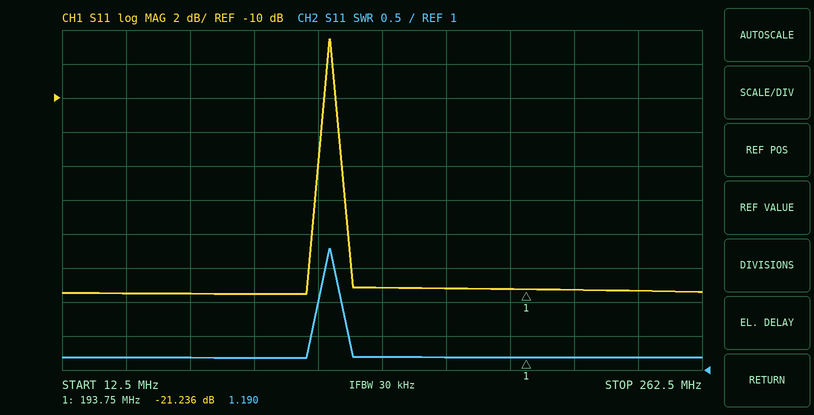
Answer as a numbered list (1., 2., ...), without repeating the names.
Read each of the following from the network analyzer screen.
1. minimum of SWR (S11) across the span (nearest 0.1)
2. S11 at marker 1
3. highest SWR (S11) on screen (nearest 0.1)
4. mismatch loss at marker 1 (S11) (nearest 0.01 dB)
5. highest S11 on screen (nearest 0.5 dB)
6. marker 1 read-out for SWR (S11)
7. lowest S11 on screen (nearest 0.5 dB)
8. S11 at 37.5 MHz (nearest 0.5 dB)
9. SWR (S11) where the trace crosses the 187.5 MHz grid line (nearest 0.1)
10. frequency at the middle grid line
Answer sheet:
1. 1.2
2. -21.236 dB
3. 2.8
4. 0.03 dB
5. -6.5 dB
6. 1.190
7. -21.5 dB
8. -21.5 dB
9. 1.2
10. 137.5 MHz
